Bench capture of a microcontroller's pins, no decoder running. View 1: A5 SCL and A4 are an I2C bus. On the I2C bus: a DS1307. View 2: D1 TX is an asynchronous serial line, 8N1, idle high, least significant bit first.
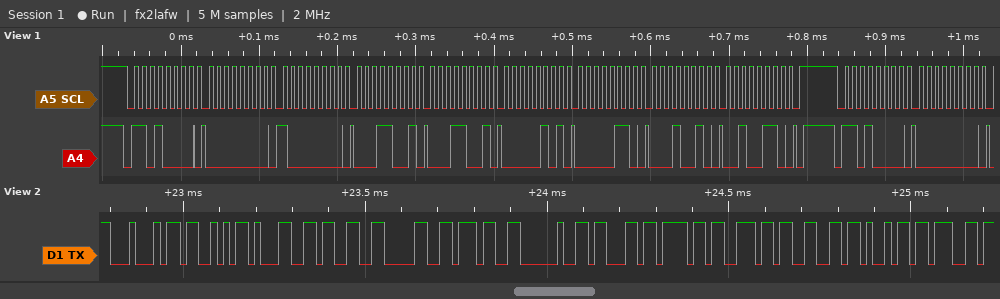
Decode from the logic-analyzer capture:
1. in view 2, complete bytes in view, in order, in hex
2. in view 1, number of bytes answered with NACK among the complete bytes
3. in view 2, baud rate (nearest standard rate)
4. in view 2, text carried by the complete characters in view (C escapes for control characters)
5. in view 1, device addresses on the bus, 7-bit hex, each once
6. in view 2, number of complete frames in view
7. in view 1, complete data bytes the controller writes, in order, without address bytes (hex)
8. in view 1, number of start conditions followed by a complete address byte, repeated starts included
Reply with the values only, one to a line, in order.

0x44 0x53 0x31 0x33 0x30 0x37 0x20 0x63 0x6F 0x6E 0x66 0x69 0x67
0
57600 baud
"DS1307 config"
0x68
13
00 80 19 19 05 06 12 26 00
2
